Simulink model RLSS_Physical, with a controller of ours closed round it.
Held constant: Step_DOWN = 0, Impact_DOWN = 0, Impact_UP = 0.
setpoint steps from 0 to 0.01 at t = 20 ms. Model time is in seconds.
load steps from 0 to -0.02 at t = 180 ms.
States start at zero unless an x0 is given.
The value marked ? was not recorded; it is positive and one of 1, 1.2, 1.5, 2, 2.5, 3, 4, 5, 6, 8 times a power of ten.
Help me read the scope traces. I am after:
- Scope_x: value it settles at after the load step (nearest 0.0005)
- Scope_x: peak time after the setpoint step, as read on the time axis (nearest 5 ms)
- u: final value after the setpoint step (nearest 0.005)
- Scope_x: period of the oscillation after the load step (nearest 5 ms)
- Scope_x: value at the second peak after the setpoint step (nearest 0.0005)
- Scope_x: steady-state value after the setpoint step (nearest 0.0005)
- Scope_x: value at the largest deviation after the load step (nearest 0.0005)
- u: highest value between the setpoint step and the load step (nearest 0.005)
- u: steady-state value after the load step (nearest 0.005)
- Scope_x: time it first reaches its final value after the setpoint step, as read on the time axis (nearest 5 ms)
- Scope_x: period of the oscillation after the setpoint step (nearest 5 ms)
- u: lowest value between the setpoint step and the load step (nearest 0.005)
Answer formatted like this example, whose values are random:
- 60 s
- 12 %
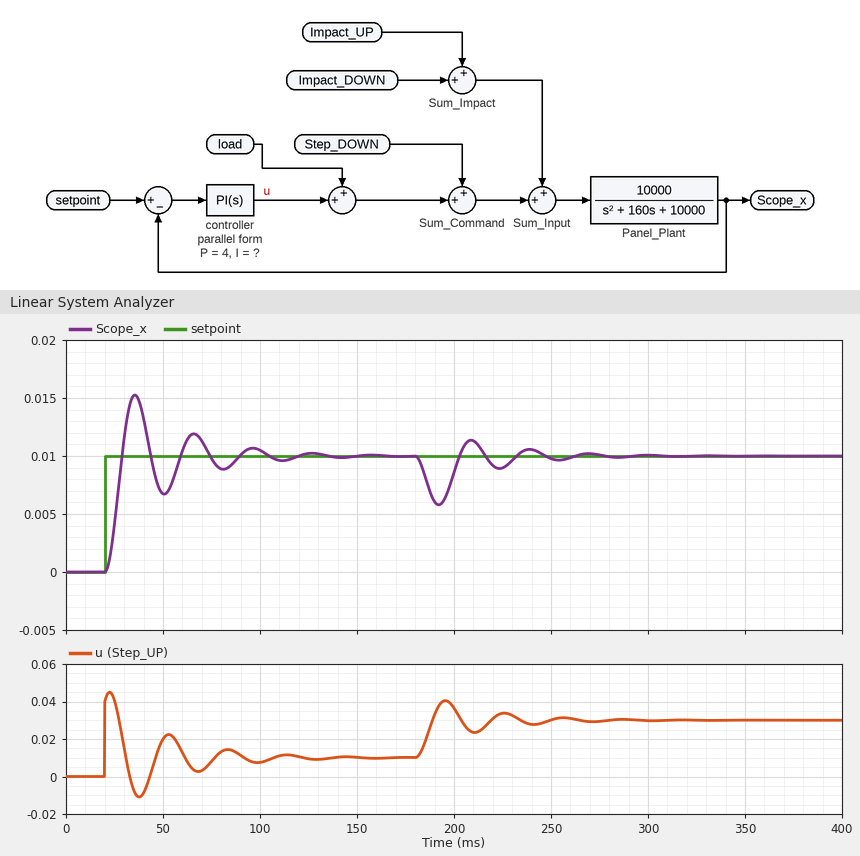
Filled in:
- 0.0100
- 35 ms
- 0.010
- 30 ms
- 0.0120
- 0.0100
- 0.0060
- 0.045
- 0.030
- 30 ms
- 30 ms
- -0.010
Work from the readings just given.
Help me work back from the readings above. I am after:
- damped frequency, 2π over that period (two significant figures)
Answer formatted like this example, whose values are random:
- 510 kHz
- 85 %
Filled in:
- 0.21 rad/ms
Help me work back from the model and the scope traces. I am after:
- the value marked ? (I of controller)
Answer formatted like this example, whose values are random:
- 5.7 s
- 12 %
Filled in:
- 400
